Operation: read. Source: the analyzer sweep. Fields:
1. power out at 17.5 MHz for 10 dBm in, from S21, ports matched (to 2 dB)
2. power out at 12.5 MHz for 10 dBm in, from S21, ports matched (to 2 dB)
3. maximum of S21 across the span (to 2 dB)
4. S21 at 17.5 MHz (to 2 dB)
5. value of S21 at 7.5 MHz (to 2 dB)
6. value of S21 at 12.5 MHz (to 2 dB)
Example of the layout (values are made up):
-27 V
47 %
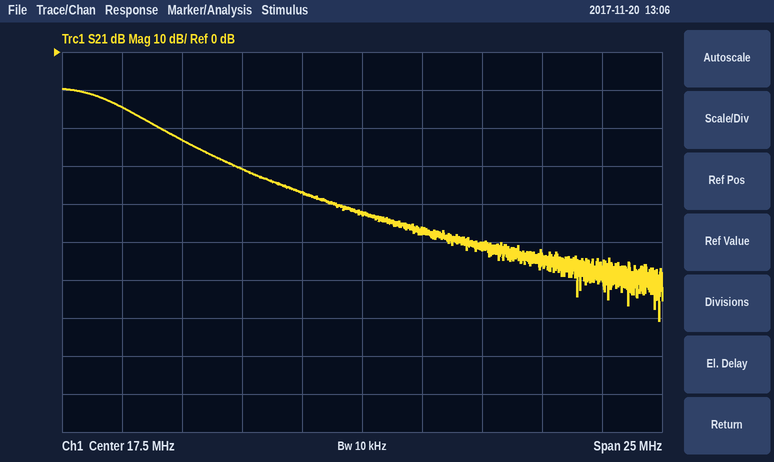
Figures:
-32 dBm
-20 dBm
-10 dB
-42 dB
-14 dB
-30 dB
